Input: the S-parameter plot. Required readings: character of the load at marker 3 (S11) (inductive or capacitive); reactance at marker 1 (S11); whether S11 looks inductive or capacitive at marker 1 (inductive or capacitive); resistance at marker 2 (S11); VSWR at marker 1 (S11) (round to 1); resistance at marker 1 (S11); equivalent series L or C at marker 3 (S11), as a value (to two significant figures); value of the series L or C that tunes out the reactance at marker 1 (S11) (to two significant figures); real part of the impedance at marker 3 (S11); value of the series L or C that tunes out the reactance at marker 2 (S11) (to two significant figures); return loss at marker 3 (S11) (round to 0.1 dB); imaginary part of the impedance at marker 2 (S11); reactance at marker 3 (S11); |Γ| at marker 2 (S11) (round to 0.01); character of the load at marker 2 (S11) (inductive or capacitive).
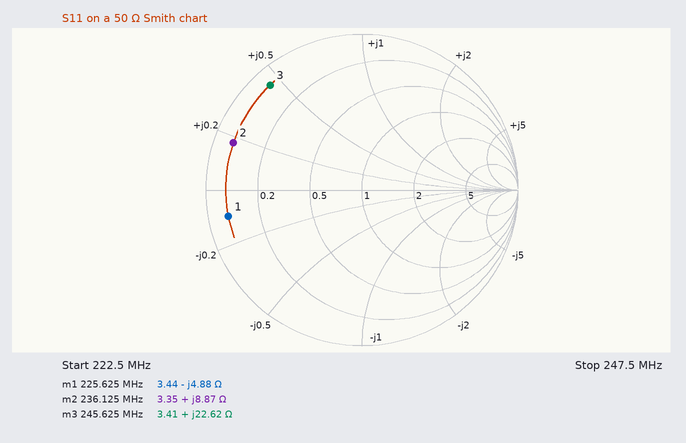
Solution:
inductive
-4.88 Ω
capacitive
3.35 Ω
15
3.44 Ω
15 nH
3.4 nH
3.41 Ω
76 pF
1.0 dB
+8.87 Ω
+22.62 Ω
0.88
inductive
